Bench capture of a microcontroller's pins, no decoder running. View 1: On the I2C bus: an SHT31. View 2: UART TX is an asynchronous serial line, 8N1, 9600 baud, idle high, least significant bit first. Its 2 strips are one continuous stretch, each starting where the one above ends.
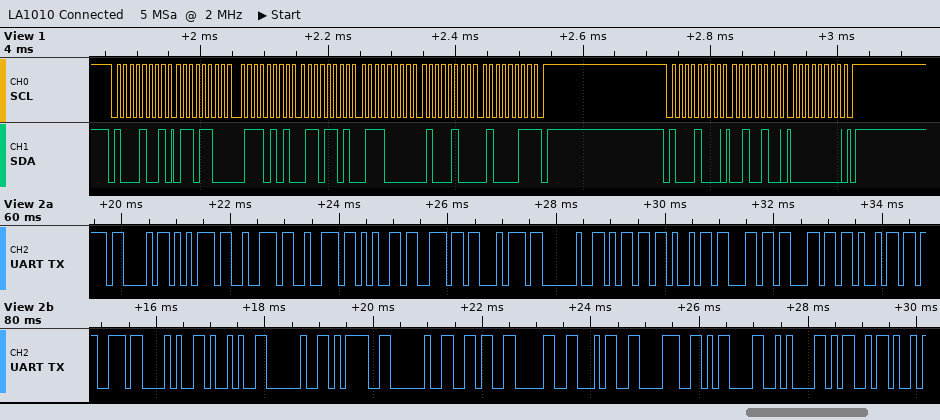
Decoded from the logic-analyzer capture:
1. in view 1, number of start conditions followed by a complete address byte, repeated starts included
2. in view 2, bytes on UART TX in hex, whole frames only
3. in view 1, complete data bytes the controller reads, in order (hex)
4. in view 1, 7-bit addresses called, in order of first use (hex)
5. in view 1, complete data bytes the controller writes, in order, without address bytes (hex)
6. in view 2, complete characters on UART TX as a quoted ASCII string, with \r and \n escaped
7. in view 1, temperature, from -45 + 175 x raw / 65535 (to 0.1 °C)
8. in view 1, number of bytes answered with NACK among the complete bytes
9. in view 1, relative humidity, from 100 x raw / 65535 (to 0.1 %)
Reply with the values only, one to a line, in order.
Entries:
2
43 75 72 72 65 6E 74 20 6D 69 6C 6C 69 73 28 29 20 3D 20 36 30 34 38 0D 0A 4D
6C 75 6D 70 44 43
0x44
24 00
"Current millis() = 6048\r\nM"
29.1 °C
1
43.9 %
